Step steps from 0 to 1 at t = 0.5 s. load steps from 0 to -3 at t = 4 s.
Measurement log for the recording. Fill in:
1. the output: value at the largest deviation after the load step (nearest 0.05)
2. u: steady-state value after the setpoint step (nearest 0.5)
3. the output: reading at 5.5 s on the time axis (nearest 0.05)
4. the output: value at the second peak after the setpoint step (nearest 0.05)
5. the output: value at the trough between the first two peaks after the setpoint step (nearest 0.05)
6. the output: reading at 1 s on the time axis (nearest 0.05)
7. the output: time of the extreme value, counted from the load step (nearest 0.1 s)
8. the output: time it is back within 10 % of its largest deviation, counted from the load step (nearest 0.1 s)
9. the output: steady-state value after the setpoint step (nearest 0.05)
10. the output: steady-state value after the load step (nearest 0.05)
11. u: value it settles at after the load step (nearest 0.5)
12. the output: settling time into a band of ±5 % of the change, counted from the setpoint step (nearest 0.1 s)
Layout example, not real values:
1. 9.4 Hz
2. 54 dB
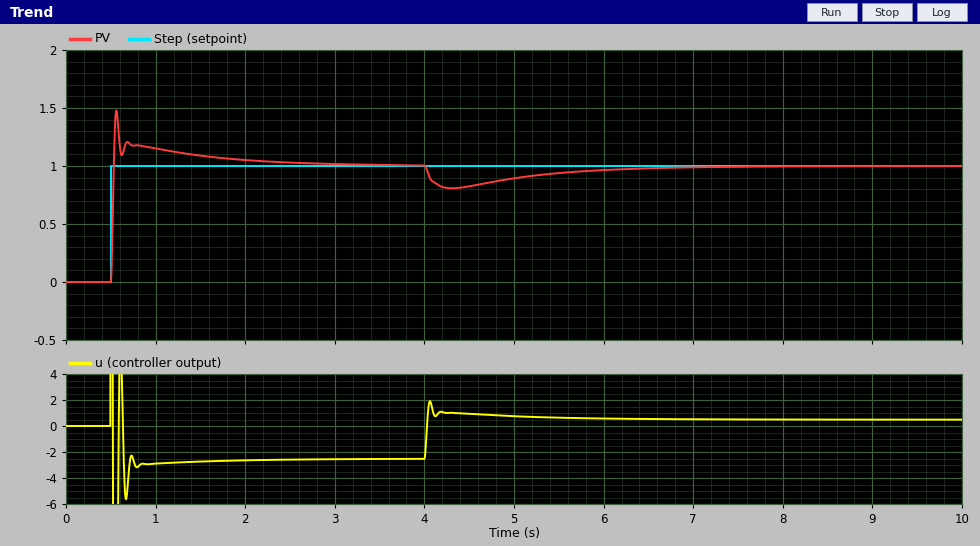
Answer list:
1. 0.80
2. -2.5
3. 0.95
4. 1.20
5. 1.10
6. 1.15
7. 0.3 s
8. 2.5 s
9. 1.00
10. 1.00
11. 0.5
12. 1.5 s
